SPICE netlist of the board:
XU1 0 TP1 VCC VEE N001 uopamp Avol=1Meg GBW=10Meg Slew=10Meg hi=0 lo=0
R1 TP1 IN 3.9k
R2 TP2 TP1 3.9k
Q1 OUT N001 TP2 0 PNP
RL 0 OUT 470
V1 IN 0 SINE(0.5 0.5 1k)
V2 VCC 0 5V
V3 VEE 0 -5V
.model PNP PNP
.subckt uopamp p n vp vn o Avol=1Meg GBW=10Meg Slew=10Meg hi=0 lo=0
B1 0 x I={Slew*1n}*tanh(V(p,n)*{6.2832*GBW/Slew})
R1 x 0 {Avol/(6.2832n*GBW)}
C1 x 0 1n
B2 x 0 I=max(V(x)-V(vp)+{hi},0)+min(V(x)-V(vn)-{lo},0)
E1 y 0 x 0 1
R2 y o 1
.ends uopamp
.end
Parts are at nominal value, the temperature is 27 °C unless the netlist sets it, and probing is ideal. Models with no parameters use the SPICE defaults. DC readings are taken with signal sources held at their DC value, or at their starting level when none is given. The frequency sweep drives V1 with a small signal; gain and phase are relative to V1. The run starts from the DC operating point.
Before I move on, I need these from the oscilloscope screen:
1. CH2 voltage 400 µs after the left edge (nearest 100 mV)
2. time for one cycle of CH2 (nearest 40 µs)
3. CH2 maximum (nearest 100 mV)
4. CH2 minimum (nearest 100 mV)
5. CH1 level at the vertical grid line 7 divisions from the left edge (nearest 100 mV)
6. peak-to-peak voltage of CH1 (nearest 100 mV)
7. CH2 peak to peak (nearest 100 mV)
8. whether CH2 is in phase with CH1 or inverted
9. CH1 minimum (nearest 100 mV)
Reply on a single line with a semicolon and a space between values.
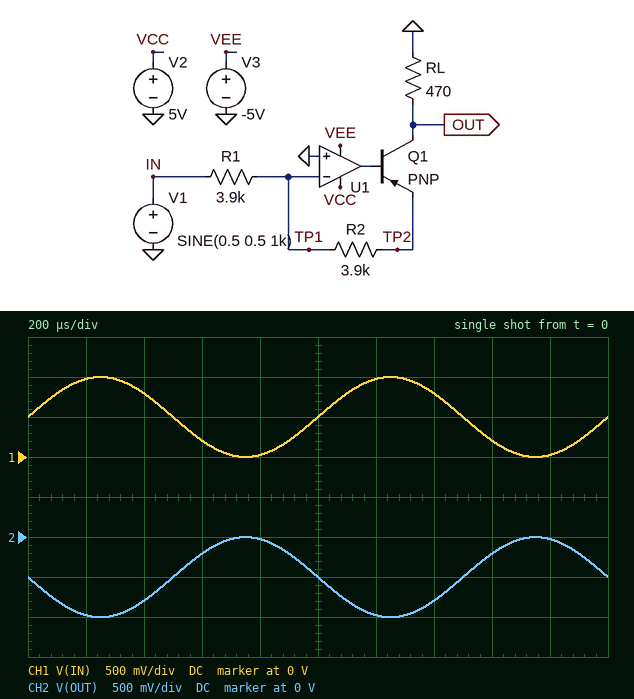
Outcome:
-800 mV; 1.00 ms; 0 V; -1.0 V; 800 mV; 1.0 V; 1.0 V; inverted; 0 V
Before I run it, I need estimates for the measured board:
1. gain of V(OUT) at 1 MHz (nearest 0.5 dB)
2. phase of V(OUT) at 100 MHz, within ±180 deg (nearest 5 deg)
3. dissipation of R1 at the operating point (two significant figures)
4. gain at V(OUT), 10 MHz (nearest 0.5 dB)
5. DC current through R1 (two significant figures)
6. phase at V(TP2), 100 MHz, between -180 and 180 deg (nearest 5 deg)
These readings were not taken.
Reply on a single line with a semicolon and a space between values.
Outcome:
0 dB; 90 deg; 64 µW; -7.5 dB; 130 µA; 85 deg
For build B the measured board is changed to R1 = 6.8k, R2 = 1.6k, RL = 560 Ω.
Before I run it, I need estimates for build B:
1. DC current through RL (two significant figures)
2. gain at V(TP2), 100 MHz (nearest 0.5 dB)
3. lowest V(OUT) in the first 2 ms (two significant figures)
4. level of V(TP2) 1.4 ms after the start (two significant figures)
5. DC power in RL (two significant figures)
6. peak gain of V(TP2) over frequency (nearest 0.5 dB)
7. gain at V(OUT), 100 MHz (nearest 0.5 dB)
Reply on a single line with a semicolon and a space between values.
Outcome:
220 µA; -33.0 dB; -240 mV; -190 mV; 27 µW; -12.5 dB; -34.5 dB
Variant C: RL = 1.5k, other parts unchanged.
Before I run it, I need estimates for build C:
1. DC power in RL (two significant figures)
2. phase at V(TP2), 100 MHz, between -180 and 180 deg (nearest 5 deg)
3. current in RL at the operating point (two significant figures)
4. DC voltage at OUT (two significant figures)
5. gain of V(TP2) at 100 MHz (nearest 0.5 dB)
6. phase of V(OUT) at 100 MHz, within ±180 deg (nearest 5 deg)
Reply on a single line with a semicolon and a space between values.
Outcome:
170 µW; 80 deg; 340 µA; -510 mV; -26.0 dB; 85 deg
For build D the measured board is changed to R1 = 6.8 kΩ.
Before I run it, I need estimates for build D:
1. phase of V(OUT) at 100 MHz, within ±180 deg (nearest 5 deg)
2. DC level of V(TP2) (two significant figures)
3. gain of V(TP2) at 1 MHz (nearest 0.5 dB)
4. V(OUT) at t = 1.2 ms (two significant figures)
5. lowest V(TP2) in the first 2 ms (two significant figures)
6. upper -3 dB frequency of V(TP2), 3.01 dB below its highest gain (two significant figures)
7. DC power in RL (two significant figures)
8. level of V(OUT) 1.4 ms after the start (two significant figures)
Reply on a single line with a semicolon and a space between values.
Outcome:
90 deg; -290 mV; -5.0 dB; -560 mV; -570 mV; 5.9 MHz; 180 µW; -460 mV
